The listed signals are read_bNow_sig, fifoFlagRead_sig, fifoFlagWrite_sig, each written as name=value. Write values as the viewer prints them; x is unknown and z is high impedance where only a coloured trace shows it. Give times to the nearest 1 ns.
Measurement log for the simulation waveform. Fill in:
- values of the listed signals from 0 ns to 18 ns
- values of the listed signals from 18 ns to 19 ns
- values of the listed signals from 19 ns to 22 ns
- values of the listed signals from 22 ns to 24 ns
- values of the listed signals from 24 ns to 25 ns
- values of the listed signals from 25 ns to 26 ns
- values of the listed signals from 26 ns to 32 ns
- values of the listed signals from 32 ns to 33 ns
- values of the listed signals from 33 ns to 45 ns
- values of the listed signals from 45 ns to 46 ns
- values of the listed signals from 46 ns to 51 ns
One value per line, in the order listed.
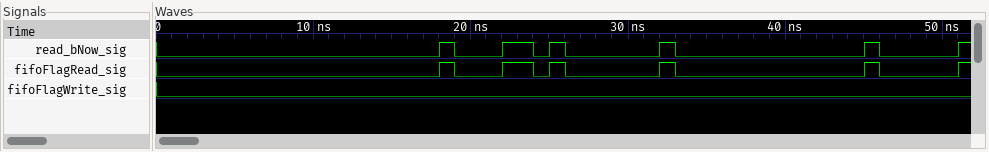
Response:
read_bNow_sig=0, fifoFlagRead_sig=0, fifoFlagWrite_sig=0
read_bNow_sig=1, fifoFlagRead_sig=1, fifoFlagWrite_sig=0
read_bNow_sig=0, fifoFlagRead_sig=0, fifoFlagWrite_sig=0
read_bNow_sig=1, fifoFlagRead_sig=1, fifoFlagWrite_sig=0
read_bNow_sig=0, fifoFlagRead_sig=0, fifoFlagWrite_sig=0
read_bNow_sig=1, fifoFlagRead_sig=1, fifoFlagWrite_sig=0
read_bNow_sig=0, fifoFlagRead_sig=0, fifoFlagWrite_sig=0
read_bNow_sig=1, fifoFlagRead_sig=1, fifoFlagWrite_sig=0
read_bNow_sig=0, fifoFlagRead_sig=0, fifoFlagWrite_sig=0
read_bNow_sig=1, fifoFlagRead_sig=1, fifoFlagWrite_sig=0
read_bNow_sig=0, fifoFlagRead_sig=0, fifoFlagWrite_sig=0
